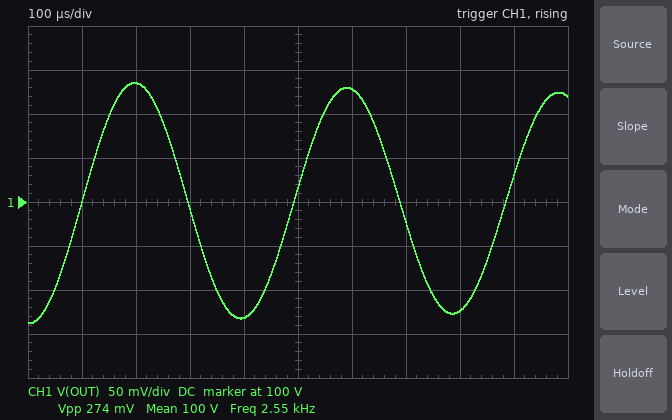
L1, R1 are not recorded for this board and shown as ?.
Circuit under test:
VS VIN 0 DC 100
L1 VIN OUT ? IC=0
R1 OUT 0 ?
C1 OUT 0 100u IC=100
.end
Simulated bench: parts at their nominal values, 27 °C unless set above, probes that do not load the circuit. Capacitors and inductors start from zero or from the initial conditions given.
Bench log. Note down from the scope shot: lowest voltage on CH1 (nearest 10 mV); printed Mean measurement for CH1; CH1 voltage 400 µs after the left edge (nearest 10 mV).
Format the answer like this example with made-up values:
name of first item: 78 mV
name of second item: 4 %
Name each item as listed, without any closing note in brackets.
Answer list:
lowest voltage on CH1: 99.86 V
printed Mean measurement for CH1: 100 V
CH1 voltage 400 µs after the left edge: 99.87 V
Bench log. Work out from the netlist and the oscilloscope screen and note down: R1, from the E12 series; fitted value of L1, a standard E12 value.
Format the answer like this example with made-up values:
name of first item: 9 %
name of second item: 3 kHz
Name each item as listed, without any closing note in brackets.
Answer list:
R1, from the E12 series: 47 Ω
fitted value of L1, a standard E12 value: 39 µH
